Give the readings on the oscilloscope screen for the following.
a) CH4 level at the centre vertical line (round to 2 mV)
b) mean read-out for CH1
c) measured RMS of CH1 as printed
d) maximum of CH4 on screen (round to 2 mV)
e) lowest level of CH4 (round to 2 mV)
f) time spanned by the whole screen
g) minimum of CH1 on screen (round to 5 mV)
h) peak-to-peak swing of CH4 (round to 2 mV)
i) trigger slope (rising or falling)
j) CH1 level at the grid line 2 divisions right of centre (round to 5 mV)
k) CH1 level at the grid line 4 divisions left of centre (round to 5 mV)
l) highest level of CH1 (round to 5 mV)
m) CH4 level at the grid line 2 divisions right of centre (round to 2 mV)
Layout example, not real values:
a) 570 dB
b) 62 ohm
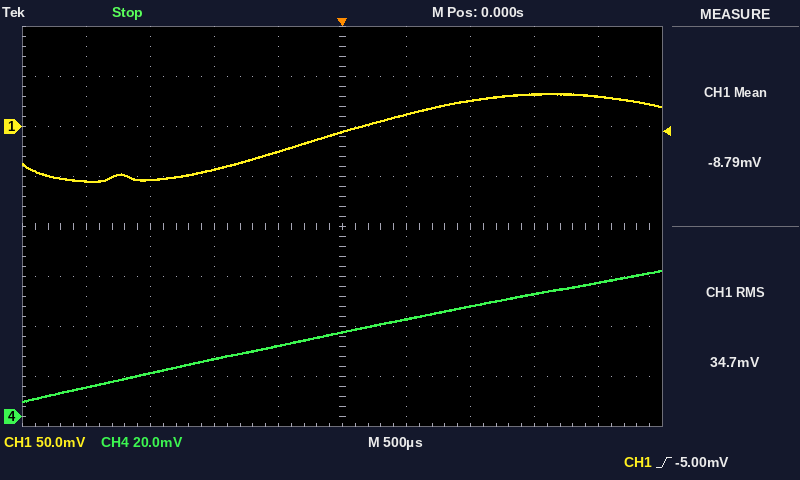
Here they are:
a) 34 mV
b) -8.79 mV
c) 34.7 mV
d) 58 mV
e) 6 mV
f) 5 ms
g) -55 mV
h) 52 mV
i) rising
j) 25 mV
k) -55 mV
l) 35 mV
m) 44 mV
